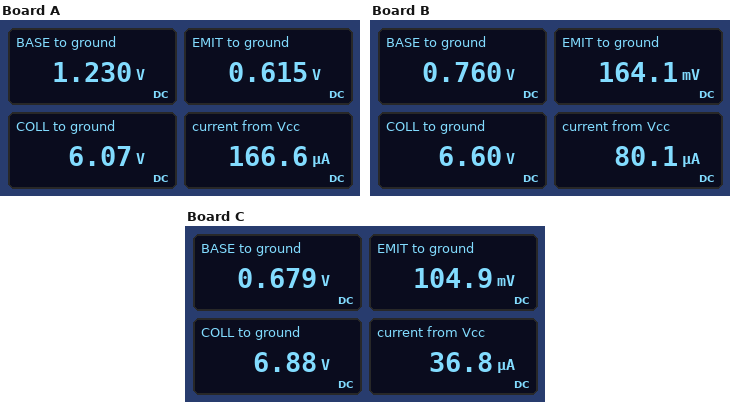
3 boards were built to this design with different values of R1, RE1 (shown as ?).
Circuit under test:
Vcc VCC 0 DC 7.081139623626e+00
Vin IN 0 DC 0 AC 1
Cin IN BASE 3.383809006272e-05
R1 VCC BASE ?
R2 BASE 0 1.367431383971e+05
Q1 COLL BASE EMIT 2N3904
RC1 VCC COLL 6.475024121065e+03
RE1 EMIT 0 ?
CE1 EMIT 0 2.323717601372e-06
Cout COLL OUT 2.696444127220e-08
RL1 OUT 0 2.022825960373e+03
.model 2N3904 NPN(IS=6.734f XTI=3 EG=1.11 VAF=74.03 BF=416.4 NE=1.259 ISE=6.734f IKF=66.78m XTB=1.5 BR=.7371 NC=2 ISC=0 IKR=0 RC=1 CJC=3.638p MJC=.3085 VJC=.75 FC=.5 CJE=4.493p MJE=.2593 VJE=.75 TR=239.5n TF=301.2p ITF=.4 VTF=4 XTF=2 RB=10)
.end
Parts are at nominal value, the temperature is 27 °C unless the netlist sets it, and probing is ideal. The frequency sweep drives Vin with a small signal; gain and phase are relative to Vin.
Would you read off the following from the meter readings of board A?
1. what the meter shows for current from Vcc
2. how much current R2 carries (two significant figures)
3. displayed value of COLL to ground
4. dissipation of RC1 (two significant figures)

166.6 µA
9.0 µA
6.07 V
160 µW
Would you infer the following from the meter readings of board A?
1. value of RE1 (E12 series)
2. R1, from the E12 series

3.9 kΩ
560 kΩ
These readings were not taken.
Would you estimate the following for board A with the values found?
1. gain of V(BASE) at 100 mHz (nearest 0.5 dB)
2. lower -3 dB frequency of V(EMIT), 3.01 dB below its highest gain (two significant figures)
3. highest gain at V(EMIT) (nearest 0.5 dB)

-1.0 dB
52 mHz
-0.5 dB
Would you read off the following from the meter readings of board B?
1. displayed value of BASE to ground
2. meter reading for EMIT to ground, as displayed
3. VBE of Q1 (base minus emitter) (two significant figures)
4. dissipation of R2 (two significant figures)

0.760 V
164.1 mV
600 mV
4.2 µW
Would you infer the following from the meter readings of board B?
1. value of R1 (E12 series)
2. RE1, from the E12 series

1 MΩ
2.2 kΩ
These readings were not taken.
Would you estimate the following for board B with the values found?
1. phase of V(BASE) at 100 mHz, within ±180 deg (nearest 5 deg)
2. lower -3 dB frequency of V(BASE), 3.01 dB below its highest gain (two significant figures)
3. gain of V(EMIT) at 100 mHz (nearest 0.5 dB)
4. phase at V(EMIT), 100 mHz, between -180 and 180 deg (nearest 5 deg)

30 deg
55 mHz
-2.5 dB
30 deg
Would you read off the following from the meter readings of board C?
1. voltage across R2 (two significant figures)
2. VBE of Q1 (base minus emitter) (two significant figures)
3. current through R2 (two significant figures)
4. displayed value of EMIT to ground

680 mV
570 mV
5.0 µA
104.9 mV
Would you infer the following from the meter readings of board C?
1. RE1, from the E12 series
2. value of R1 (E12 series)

3.3 kΩ
1.2 MΩ
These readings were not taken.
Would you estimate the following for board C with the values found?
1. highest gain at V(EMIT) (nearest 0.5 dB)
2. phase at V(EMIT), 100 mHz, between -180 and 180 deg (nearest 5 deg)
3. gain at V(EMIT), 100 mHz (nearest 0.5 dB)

-2.0 dB
25 deg
-3.0 dB
